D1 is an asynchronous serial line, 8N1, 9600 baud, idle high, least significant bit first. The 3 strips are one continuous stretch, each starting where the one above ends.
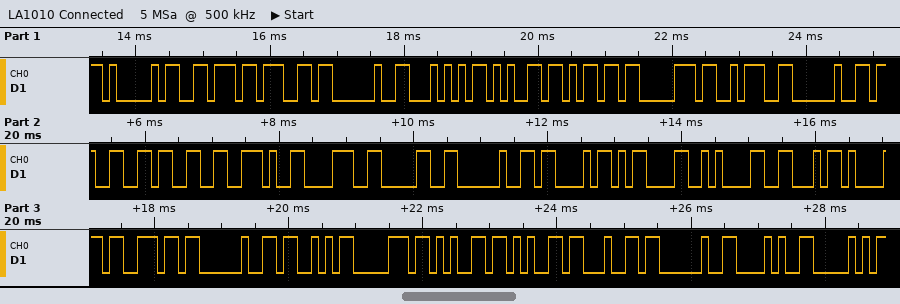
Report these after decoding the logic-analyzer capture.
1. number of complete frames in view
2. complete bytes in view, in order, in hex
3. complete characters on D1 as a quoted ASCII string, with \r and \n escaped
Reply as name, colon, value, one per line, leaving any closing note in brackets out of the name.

number of complete frames in view: 31
complete bytes in view, in order, in hex: 0x41 0x76 0x67 0x20 0x54 0x65 0x6D 0x70 0x3A 0x20 0x33 0x33 0x2E 0x38 0x30 0x20 0x43 0x0D 0x0A 0x46 0x61 0x6E 0x20 0x53 0x70 0x65 0x65 0x64 0x20 0x28 0x50
complete characters on D1 as a quoted ASCII string, with \r and \n escaped: "Avg Temp: 33.80 C\r\nFan Speed (P"
